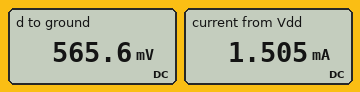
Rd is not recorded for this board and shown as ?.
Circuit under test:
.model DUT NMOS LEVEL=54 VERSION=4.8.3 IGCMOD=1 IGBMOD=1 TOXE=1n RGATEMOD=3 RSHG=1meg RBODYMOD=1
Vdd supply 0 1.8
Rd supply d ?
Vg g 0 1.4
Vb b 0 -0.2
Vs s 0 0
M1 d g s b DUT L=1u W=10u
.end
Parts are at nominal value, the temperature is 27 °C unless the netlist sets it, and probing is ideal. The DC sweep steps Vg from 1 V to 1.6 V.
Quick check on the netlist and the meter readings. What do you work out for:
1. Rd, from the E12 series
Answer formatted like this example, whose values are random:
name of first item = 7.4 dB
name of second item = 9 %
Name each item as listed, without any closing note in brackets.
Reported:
Rd, from the E12 series = 820 Ω
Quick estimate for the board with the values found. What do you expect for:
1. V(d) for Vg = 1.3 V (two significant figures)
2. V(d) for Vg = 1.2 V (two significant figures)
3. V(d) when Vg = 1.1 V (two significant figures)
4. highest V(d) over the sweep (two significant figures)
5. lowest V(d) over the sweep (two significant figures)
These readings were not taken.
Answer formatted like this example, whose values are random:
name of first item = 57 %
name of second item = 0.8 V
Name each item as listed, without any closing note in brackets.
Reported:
V(d) for Vg = 1.3 V = 600 mV
V(d) for Vg = 1.2 V = 640 mV
V(d) when Vg = 1.1 V = 680 mV
highest V(d) over the sweep = 730 mV
lowest V(d) over the sweep = 510 mV
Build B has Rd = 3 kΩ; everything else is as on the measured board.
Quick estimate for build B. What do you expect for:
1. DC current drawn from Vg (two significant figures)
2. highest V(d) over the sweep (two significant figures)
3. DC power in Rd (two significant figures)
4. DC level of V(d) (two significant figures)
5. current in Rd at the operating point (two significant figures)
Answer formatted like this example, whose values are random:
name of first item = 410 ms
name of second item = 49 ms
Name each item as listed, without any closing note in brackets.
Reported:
DC current drawn from Vg = 310 nA
highest V(d) over the sweep = 130 mV
DC power in Rd = 940 µW
DC level of V(d) = 120 mV
current in Rd at the operating point = 560 µA
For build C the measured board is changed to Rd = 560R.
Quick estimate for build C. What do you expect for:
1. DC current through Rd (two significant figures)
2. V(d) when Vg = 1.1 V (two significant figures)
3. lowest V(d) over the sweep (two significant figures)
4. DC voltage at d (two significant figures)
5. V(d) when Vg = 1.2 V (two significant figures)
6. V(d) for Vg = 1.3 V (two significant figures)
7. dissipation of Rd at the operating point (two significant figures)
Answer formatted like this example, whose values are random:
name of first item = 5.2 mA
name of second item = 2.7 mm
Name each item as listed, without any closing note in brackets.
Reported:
DC current through Rd = 1.6 mA
V(d) when Vg = 1.1 V = 1.0 V
lowest V(d) over the sweep = 870 mV
DC voltage at d = 920 mV
V(d) when Vg = 1.2 V = 980 mV
V(d) for Vg = 1.3 V = 950 mV
dissipation of Rd at the operating point = 1.4 mW
